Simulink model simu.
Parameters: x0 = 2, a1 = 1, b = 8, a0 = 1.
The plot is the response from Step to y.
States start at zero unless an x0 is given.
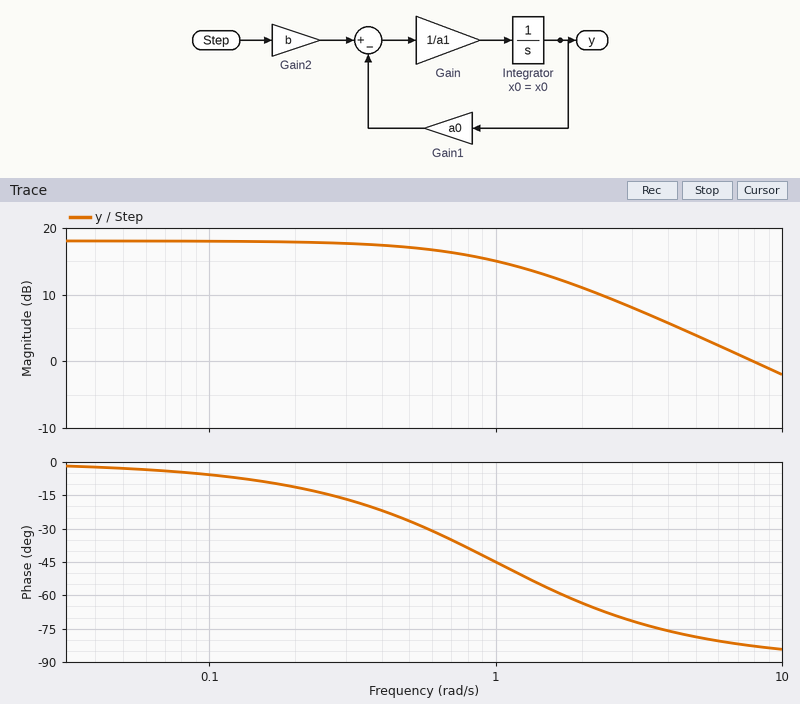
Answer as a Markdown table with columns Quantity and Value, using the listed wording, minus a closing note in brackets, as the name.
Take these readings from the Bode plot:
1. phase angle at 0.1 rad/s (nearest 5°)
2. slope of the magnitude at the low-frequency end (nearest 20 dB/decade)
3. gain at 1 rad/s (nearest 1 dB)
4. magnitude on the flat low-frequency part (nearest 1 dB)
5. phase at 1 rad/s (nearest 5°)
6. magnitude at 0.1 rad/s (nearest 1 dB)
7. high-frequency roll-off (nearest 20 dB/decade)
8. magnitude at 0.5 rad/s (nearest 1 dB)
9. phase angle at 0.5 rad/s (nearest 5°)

| Quantity | Value |
|---|---|
| phase angle at 0.1 rad/s | -5° |
| slope of the magnitude at the low-frequency end | 0 dB/decade |
| gain at 1 rad/s | 15 dB |
| magnitude on the flat low-frequency part | 18 dB |
| phase at 1 rad/s | -45° |
| magnitude at 0.1 rad/s | 18 dB |
| high-frequency roll-off | -20 dB/decade |
| magnitude at 0.5 rad/s | 17 dB |
| phase angle at 0.5 rad/s | -25° |
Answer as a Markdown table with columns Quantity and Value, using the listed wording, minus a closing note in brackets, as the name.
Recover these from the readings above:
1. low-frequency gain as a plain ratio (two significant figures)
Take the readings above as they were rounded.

| Quantity | Value |
|---|---|
| low-frequency gain as a plain ratio | 7.9 |
